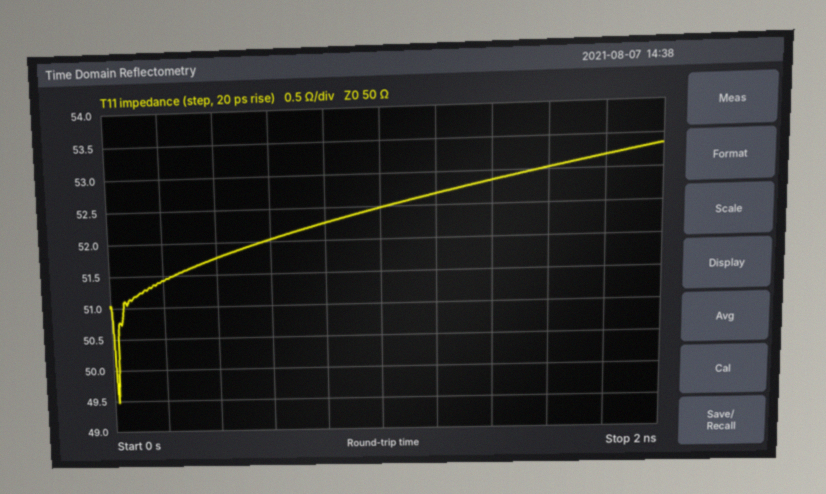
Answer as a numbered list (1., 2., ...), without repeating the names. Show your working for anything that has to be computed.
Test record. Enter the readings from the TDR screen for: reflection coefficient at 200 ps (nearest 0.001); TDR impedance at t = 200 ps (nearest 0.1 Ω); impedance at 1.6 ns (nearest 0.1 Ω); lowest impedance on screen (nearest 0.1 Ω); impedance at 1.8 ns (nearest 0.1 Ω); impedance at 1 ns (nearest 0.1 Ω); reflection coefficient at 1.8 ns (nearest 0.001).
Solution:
1. (51.4 − 50)/(51.4 + 50) ≈ +0.014
2. 51.4 Ω
3. 53.0 Ω
4. 49.5 Ω
5. 53.2 Ω
6. 52.5 Ω
7. (53.2 − 50)/(53.2 + 50) ≈ +0.031
